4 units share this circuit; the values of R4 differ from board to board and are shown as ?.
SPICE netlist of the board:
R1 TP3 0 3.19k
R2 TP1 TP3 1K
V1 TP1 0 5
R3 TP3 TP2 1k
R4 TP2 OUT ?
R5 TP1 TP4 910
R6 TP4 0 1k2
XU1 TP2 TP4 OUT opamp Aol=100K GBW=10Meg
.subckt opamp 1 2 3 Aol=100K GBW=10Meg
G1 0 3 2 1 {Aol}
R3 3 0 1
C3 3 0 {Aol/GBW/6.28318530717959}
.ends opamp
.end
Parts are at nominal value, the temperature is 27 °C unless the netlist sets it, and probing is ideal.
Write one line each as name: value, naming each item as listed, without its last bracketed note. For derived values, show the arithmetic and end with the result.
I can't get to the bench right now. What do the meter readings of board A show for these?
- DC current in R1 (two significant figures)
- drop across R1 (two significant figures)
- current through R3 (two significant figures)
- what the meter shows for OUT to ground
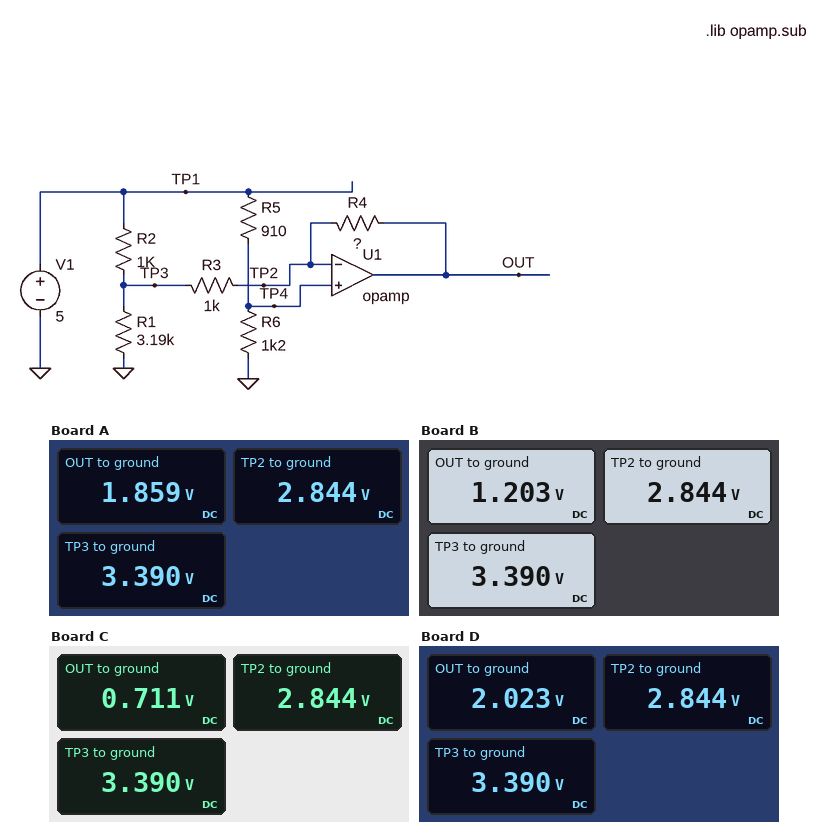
DC current in R1: (3.39 V) / 3.19 kΩ = 1.1 mA
drop across R1: 3.39 V = 3.4 V
current through R3: (3.39 V - 2.844 V) / 1 kΩ = 550 µA
what the meter shows for OUT to ground: 1.859 V
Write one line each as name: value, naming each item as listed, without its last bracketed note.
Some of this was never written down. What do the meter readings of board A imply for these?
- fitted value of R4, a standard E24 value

fitted value of R4, a standard E24 value: 1.8 kΩ
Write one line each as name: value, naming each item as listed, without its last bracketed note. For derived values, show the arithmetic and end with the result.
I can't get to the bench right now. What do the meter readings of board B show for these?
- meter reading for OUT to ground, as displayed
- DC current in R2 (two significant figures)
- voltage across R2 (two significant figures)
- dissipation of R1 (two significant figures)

meter reading for OUT to ground, as displayed: 1.203 V
DC current in R2: (5 V - 3.39 V) / 1 kΩ = 1.6 mA
voltage across R2: 5 V - 3.39 V = 1.6 V
dissipation of R1: (3.39 V)^2 / 3.19 kΩ = 3.6 mW
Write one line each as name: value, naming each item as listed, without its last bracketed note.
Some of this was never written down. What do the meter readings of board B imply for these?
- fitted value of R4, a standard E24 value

fitted value of R4, a standard E24 value: 3 kΩ
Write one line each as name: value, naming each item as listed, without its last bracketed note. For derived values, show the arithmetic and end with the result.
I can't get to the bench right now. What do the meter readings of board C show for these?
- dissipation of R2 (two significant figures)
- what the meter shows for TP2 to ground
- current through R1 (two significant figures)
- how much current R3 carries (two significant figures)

dissipation of R2: (5 V - 3.39 V)^2 / 1 kΩ = 2.6 mW
what the meter shows for TP2 to ground: 2.844 V
current through R1: (3.39 V) / 3.19 kΩ = 1.1 mA
how much current R3 carries: (3.39 V - 2.844 V) / 1 kΩ = 550 µA
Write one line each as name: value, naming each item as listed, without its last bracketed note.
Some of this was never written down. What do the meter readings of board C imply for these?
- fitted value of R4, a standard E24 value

fitted value of R4, a standard E24 value: 3.9 kΩ
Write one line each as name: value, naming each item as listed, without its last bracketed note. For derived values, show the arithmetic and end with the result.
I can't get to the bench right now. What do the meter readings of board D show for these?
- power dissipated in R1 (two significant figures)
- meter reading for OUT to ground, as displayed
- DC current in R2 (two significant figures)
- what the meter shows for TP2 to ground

power dissipated in R1: (3.39 V)^2 / 3.19 kΩ = 3.6 mW
meter reading for OUT to ground, as displayed: 2.023 V
DC current in R2: (5 V - 3.39 V) / 1 kΩ = 1.6 mA
what the meter shows for TP2 to ground: 2.844 V
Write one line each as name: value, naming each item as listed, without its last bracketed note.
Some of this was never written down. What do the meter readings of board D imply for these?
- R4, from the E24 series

R4, from the E24 series: 1.5 kΩ
